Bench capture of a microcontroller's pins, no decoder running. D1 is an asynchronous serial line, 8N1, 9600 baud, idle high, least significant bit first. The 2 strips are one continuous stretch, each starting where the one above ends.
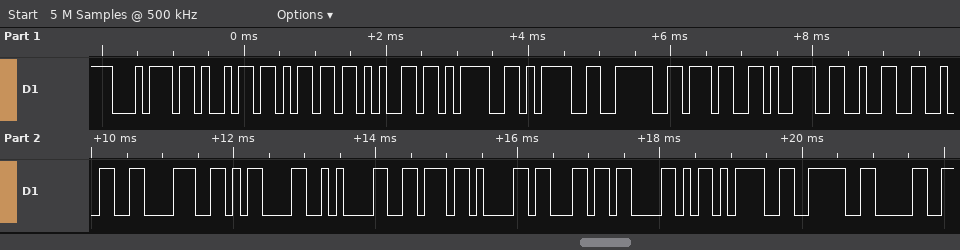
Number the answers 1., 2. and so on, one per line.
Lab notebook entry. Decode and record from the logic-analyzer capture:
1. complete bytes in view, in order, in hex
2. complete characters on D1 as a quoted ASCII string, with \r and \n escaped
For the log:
1. 74 69 6D 65 3D 3D 3E 37 39 32 32 38 0D 0A 76 61 6C 58 3D 3E 30
2. "time==>79228\r\nvalX=>0"
